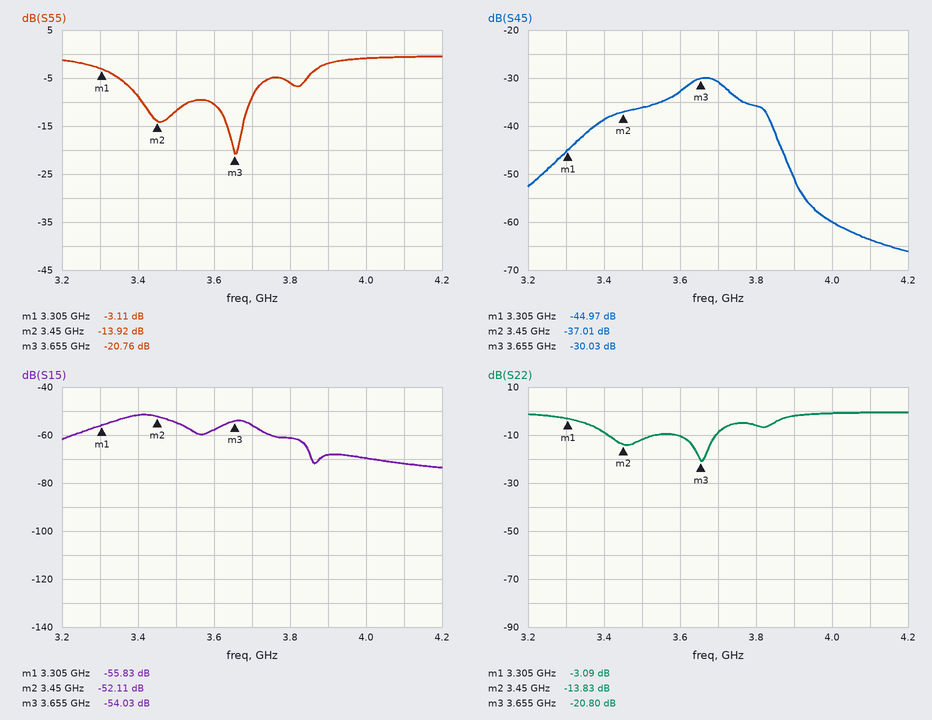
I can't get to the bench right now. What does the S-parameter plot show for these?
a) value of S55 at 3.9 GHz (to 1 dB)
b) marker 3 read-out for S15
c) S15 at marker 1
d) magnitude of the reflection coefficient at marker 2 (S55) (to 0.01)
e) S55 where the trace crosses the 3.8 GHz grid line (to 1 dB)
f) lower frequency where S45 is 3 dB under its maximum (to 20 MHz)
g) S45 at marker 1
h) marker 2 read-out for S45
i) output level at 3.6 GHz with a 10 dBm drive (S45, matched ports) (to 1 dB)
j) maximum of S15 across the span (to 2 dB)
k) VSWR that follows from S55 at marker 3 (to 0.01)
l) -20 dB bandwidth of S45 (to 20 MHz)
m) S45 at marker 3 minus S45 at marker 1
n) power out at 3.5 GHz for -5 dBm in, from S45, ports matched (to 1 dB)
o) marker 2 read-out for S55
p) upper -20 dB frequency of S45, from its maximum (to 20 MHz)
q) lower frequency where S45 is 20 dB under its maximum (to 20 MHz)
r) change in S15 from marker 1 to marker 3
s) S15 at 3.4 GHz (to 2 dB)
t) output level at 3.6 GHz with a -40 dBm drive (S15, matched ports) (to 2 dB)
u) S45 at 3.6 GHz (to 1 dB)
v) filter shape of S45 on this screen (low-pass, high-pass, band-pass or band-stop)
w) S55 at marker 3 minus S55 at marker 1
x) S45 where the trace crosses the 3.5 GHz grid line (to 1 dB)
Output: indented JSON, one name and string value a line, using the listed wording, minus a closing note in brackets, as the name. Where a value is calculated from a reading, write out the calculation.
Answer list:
{
  "value of S55 at 3.9 GHz": "-2 dB",
  "marker 3 read-out for S15": "-54.03 dB",
  "S15 at marker 1": "-55.83 dB",
  "magnitude of the reflection coefficient at marker 2 (S55)": "10^(-13.92/20) ≈ 0.20",
  "S55 where the trace crosses the 3.8 GHz grid line": "-6 dB",
  "lower frequency where S45 is 3 dB under its maximum": "3.60 GHz",
  "S45 at marker 1": "-44.97 dB",
  "marker 2 read-out for S45": "-37.01 dB",
  "output level at 3.6 GHz with a 10 dBm drive (S45, matched ports)": "10 dBm + (-33 dB) = -23 dBm",
  "maximum of S15 across the span": "-52 dB",
  "VSWR that follows from S55 at marker 3": "(1 + 0.0916)/(1 − 0.0916) ≈ 1.20",
  "-20 dB bandwidth of S45": "3.90 GHz − 3.24 GHz = 660 MHz",
  "S45 at marker 3 minus S45 at marker 1": "-30.03 − (-44.97) = 14.94 dB",
  "power out at 3.5 GHz for -5 dBm in, from S45, ports matched": "-5 dBm + (-36 dB) = -41 dBm",
  "marker 2 read-out for S55": "-13.92 dB",
  "upper -20 dB frequency of S45, from its maximum": "3.90 GHz",
  "lower frequency where S45 is 20 dB under its maximum": "3.24 GHz",
  "change in S15 from marker 1 to marker 3": "-54.03 − (-55.83) = 1.80 dB",
  "S15 at 3.4 GHz": "-52 dB",
  "output level at 3.6 GHz with a -40 dBm drive (S15, matched ports)": "-40 dBm + (-58 dB) = -98 dBm",
  "S45 at 3.6 GHz": "-33 dB",
  "filter shape of S45 on this screen": "band-pass",
  "S55 at marker 3 minus S55 at marker 1": "-20.76 − (-3.11) = -17.65 dB",
  "S45 where the trace crosses the 3.5 GHz grid line": "-36 dB"
}
